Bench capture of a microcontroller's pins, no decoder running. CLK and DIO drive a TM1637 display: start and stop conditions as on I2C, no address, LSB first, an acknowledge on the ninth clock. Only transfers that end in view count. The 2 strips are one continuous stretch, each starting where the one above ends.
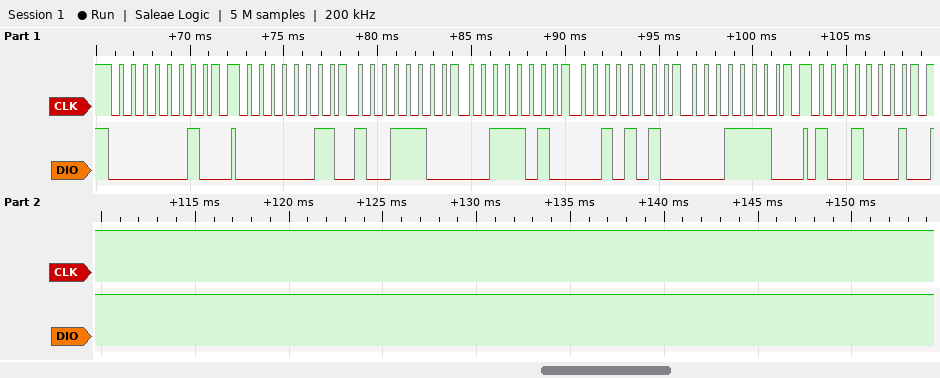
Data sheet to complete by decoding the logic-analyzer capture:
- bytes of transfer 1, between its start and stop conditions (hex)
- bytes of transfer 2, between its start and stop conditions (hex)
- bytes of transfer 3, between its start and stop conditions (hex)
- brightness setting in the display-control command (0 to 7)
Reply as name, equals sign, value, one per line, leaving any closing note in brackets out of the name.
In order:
bytes of transfer 1, between its start and stop conditions = 40
bytes of transfer 2, between its start and stop conditions = C0 39 5C 54 78
bytes of transfer 3, between its start and stop conditions = 89
brightness setting in the display-control command = 1
